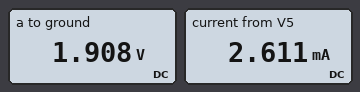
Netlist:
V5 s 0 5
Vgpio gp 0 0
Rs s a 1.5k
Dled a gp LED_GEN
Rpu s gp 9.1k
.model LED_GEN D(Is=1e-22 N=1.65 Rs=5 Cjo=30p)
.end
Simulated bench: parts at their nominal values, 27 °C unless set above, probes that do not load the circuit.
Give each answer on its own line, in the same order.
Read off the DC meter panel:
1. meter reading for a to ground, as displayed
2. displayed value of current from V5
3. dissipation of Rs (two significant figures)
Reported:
1.908 V
2.611 mA
6.4 mW
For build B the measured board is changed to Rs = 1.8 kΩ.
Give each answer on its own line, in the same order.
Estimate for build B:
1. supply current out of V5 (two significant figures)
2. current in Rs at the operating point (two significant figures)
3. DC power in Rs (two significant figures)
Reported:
2.3 mA
1.7 mA
5.3 mW
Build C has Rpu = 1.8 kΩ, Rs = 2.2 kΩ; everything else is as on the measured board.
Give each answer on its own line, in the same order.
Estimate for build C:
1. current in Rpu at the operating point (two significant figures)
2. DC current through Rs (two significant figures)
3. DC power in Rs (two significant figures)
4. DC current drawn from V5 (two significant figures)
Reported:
2.8 mA
1.4 mA
4.4 mW
4.2 mA
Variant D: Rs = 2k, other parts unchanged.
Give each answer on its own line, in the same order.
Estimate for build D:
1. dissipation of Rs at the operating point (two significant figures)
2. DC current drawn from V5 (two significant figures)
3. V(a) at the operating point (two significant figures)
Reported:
4.8 mW
2.1 mA
1.9 V
